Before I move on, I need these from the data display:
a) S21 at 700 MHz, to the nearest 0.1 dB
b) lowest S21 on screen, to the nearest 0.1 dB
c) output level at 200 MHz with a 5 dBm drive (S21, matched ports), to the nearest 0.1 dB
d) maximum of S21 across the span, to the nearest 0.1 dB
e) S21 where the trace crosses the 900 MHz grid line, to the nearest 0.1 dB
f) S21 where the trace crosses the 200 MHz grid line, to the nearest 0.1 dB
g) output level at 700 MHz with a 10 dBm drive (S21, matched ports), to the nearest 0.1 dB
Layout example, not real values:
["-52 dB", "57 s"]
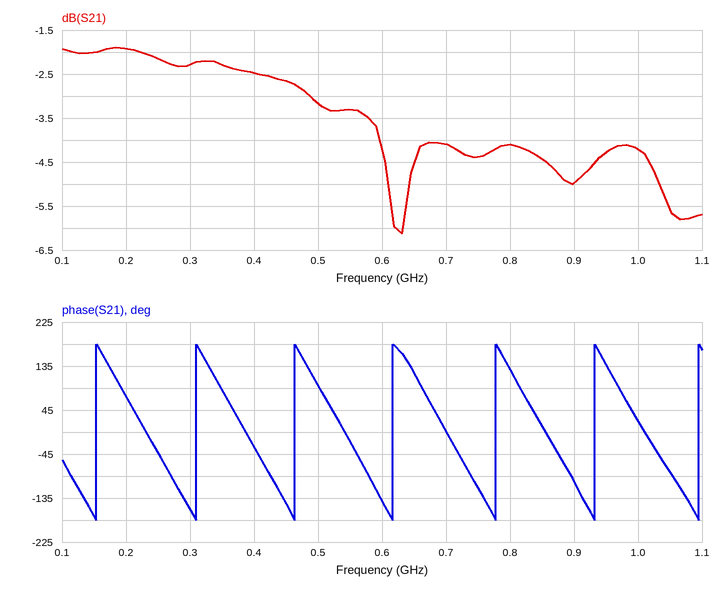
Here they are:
["-4.1 dB", "-6.1 dB", "3.1 dBm", "-1.9 dB", "-5.0 dB", "-1.9 dB", "5.9 dBm"]
